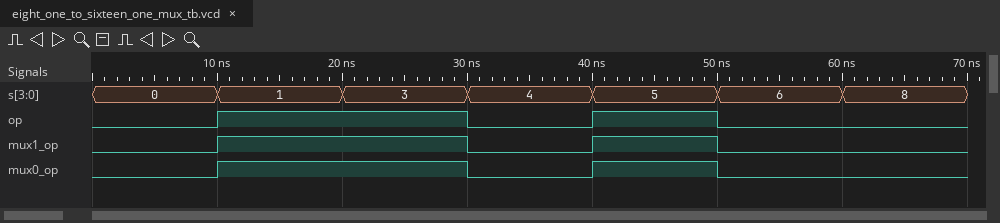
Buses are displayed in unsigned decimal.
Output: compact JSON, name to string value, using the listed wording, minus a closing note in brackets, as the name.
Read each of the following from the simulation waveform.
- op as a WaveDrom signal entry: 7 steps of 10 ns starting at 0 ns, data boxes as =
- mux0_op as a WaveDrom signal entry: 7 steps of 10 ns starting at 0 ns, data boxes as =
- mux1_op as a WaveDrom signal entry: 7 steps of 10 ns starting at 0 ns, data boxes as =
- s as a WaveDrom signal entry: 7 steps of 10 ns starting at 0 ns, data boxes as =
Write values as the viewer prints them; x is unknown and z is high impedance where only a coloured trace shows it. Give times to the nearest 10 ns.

{"op as a WaveDrom signal entry: 7 steps of 10 ns starting at 0 ns, data boxes as =": "{name: 'op', wave: '01.010.'}", "mux0_op as a WaveDrom signal entry: 7 steps of 10 ns starting at 0 ns, data boxes as =": "{name: 'mux0_op', wave: '01.010.'}", "mux1_op as a WaveDrom signal entry: 7 steps of 10 ns starting at 0 ns, data boxes as =": "{name: 'mux1_op', wave: '01.010.'}", "s as a WaveDrom signal entry: 7 steps of 10 ns starting at 0 ns, data boxes as =": "{name: 's', wave: '=======', data: '0 1 3 4 5 6 8'}"}
